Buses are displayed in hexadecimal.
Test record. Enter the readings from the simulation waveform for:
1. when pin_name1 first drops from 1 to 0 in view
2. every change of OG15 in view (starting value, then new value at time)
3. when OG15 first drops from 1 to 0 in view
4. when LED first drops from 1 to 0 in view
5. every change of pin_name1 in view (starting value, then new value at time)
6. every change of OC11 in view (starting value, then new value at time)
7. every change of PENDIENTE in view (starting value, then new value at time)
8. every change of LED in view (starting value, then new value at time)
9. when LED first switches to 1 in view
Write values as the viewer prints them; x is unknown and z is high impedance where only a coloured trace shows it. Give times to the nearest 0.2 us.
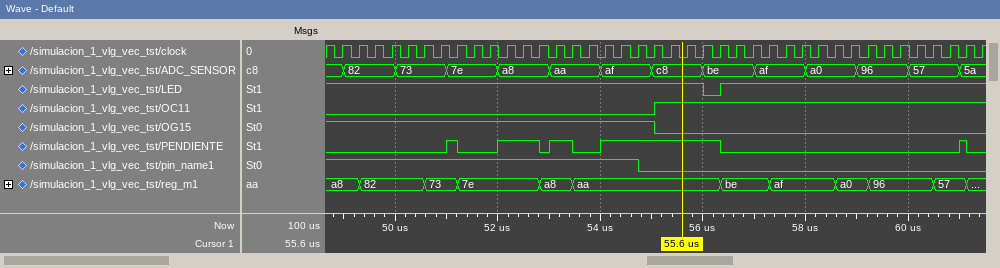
54.8 us
1, 0 at 55 us
55 us
56 us
1, 0 at 54.8 us
0, 1 at 55 us
0, 1 at 51 us, 0 at 51.2 us, 1 at 52 us, 0 at 52.8 us, 1 at 53 us, 0 at 53.4 us, 1 at 54 us, 0 at 56.4 us, 1 at 61 us, 0 at 61.2 us
1, 0 at 56 us, 1 at 56.4 us
56.4 us
